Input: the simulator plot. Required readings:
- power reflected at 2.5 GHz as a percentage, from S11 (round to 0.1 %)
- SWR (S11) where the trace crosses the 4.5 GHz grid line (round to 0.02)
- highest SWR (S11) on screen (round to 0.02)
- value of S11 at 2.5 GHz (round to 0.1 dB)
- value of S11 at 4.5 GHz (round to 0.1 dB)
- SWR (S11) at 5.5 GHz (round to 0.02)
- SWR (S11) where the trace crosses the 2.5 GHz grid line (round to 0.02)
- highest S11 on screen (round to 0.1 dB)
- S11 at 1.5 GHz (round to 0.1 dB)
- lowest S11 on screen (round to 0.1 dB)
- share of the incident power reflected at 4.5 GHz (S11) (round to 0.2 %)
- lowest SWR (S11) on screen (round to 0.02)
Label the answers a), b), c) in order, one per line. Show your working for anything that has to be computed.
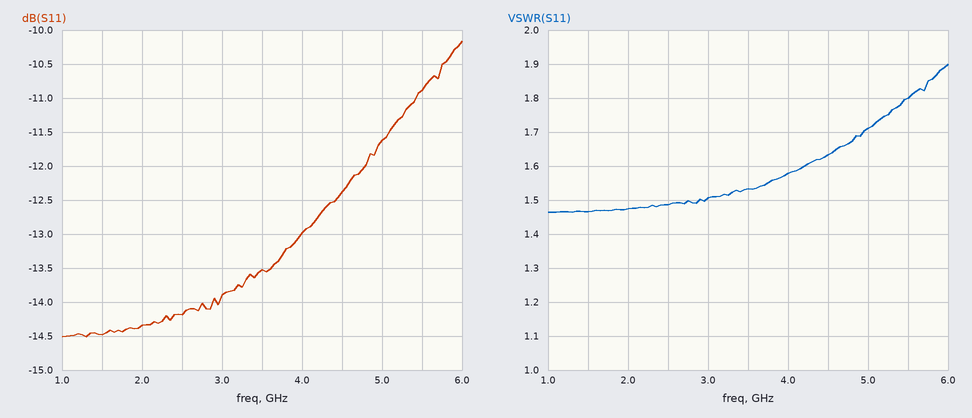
a) 10^(-14.2/10) ≈ 3.8 %
b) 1.64
c) 1.90
d) -14.2 dB
e) -12.4 dB
f) 1.80
g) 1.48
h) -10.2 dB
i) -14.5 dB
j) -14.5 dB
k) 10^(-12.4/10) ≈ 5.8 %
l) 1.46
